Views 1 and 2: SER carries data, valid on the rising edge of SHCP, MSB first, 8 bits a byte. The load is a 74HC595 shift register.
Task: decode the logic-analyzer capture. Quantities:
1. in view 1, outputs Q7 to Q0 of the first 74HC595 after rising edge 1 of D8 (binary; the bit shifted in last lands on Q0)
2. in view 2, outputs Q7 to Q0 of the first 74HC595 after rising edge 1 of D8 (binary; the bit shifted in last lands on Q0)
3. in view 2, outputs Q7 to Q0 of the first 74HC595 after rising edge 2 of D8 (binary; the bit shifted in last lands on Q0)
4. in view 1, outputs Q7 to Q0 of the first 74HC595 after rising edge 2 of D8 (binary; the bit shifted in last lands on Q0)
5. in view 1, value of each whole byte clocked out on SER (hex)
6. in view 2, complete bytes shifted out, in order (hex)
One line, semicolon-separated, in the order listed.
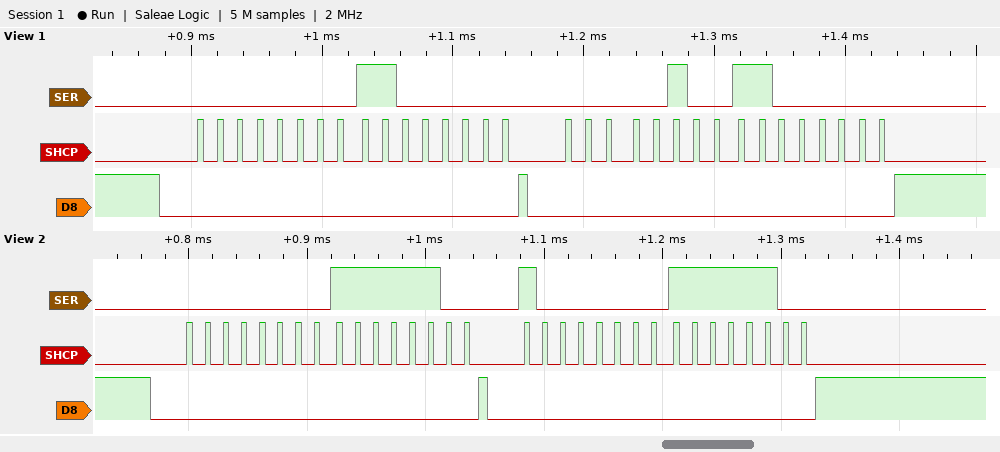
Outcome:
11000000; 11111100; 11111100; 11000000; 00 C0 04 C0; 00 FC 80 FC
